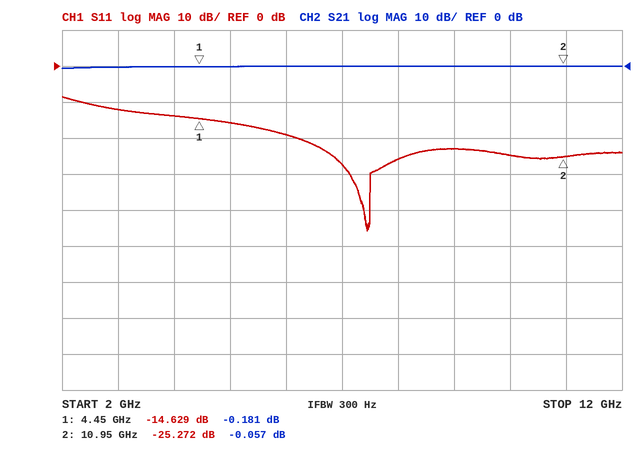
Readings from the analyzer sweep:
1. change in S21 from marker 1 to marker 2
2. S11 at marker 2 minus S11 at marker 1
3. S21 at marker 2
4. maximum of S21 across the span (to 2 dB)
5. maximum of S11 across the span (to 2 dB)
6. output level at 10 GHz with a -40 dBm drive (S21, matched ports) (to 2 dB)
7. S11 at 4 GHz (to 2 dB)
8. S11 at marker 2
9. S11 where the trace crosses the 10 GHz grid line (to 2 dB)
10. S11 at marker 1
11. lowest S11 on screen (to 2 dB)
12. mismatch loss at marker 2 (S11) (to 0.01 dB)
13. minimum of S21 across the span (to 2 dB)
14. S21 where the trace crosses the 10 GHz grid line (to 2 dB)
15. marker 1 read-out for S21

0.124 dB
-10.643 dB
-0.057 dB
0 dB
-8 dB
-40 dBm
-14 dB
-25.272 dB
-24 dB
-14.629 dB
-46 dB
0.01 dB
0 dB
0 dB
-0.181 dB
